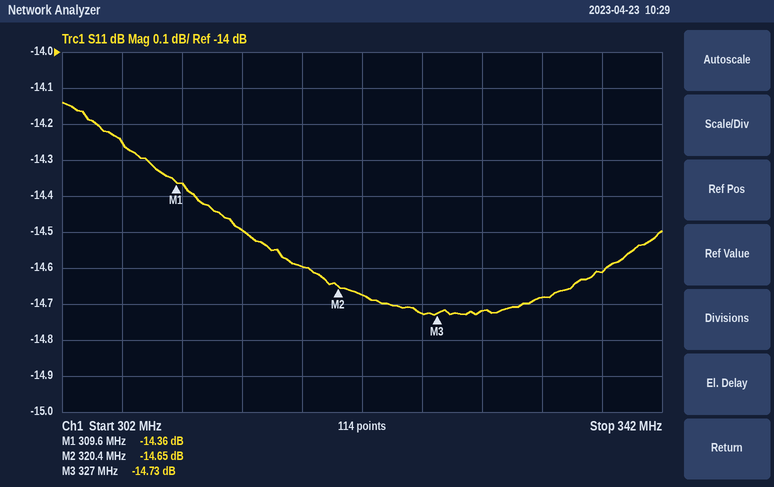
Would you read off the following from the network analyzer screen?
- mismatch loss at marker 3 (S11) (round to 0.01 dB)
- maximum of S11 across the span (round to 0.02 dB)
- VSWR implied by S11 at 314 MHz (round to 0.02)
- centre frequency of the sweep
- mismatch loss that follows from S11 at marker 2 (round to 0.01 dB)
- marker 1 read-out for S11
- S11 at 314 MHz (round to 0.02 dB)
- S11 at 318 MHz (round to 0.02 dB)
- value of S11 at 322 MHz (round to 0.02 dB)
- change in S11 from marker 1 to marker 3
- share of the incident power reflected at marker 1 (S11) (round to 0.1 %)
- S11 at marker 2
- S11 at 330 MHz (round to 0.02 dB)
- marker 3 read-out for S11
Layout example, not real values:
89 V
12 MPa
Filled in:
0.15 dB
-14.14 dB
1.46
322 MHz
0.15 dB
-14.36 dB
-14.50 dB
-14.60 dB
-14.68 dB
-0.37 dB
3.7 %
-14.65 dB
-14.72 dB
-14.73 dB
